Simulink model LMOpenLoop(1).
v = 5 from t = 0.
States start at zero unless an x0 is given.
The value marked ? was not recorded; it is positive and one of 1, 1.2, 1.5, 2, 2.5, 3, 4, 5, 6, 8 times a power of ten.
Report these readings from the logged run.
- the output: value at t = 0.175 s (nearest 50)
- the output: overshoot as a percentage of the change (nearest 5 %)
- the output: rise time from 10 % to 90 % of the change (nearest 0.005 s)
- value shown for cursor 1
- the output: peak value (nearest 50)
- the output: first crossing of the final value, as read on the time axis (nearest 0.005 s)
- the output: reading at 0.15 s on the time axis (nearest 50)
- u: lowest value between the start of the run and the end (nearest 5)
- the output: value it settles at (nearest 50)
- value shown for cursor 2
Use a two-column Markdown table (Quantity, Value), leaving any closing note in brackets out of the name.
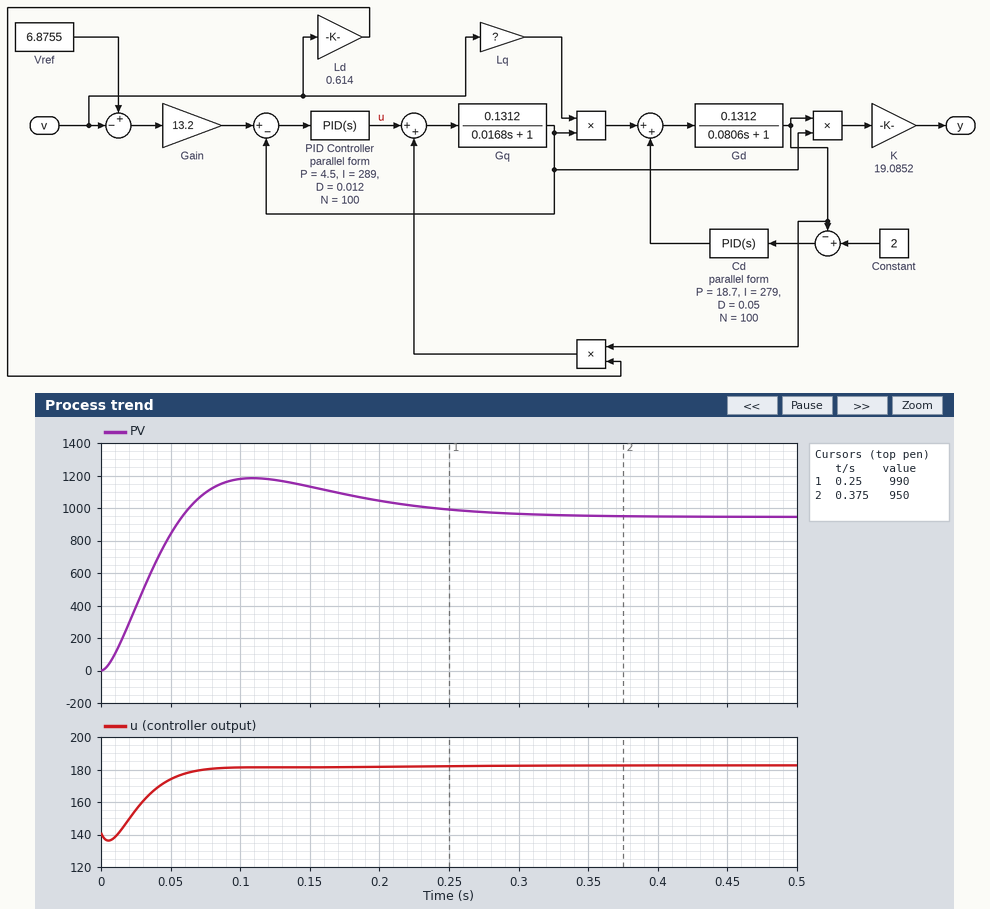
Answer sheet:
| Quantity | Value |
|---|---|
| the output: value at t = 0.175 s | 1100 |
| the output: overshoot as a percentage of the change | 25 % |
| the output: rise time from 10 % to 90 % of the change | 0.040 s |
| value shown for cursor 1 | 990 |
| the output: peak value | 1200 |
| the output: first crossing of the final value, as read on the time axis | 0.060 s |
| the output: reading at 0.15 s on the time axis | 1150 |
| u: lowest value between the start of the run and the end | 135 |
| the output: value it settles at | 950 |
| value shown for cursor 2 | 950 |
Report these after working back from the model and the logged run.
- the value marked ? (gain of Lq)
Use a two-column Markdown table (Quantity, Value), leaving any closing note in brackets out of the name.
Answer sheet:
| Quantity | Value |
|---|---|
| the value marked ? | 0.2 |
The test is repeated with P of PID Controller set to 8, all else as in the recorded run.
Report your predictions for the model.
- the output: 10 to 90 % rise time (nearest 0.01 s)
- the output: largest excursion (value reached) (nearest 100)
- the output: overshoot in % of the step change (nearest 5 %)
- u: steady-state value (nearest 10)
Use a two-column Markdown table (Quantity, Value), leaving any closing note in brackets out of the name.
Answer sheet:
| Quantity | Value |
|---|---|
| the output: 10 to 90 % rise time | 0.04 s |
| the output: largest excursion (value reached) | 1100 |
| the output: overshoot in % of the step change | 20 % |
| u: steady-state value | 180 |
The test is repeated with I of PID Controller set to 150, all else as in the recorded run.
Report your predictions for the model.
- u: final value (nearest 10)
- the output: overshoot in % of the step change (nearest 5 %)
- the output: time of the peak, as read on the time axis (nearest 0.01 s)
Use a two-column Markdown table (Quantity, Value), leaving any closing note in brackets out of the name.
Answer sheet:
| Quantity | Value |
|---|---|
| u: final value | 180 |
| the output: overshoot in % of the step change | 10 % |
| the output: time of the peak, as read on the time axis | 0.15 s |
